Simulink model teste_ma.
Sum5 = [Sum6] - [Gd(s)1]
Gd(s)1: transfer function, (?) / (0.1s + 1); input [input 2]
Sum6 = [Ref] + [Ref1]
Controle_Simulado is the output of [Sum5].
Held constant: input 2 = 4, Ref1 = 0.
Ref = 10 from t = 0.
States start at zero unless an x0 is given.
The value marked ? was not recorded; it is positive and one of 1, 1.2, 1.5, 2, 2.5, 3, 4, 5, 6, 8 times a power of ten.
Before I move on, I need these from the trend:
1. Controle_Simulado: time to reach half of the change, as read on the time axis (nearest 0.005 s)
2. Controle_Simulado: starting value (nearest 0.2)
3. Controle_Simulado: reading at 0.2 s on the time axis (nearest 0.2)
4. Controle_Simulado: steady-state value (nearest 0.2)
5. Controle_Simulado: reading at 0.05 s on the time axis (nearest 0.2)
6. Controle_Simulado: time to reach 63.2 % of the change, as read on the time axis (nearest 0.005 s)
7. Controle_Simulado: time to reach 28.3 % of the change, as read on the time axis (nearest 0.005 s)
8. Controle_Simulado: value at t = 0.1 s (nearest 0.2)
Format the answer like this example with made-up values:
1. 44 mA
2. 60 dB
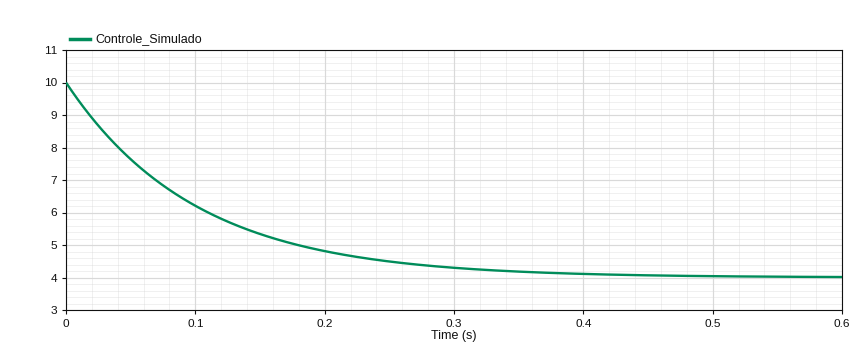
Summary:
1. 0.070 s
2. 10.0
3. 4.8
4. 4.0
5. 7.6
6. 0.100 s
7. 0.035 s
8. 6.2
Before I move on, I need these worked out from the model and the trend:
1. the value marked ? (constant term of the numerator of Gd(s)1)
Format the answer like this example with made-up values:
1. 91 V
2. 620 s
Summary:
1. 1.5
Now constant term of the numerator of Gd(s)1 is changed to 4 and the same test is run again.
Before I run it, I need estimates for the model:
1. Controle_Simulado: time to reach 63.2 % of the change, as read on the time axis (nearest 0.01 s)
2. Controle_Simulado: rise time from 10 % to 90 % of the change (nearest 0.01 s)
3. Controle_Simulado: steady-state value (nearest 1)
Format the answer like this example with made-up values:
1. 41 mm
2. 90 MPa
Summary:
1. 0.10 s
2. 0.22 s
3. -6
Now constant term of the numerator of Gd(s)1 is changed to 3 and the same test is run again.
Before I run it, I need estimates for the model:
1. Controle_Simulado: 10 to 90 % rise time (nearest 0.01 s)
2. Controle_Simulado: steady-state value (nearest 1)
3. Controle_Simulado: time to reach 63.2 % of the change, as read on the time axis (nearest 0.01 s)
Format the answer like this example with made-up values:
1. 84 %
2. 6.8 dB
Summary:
1. 0.22 s
2. -2
3. 0.10 s
